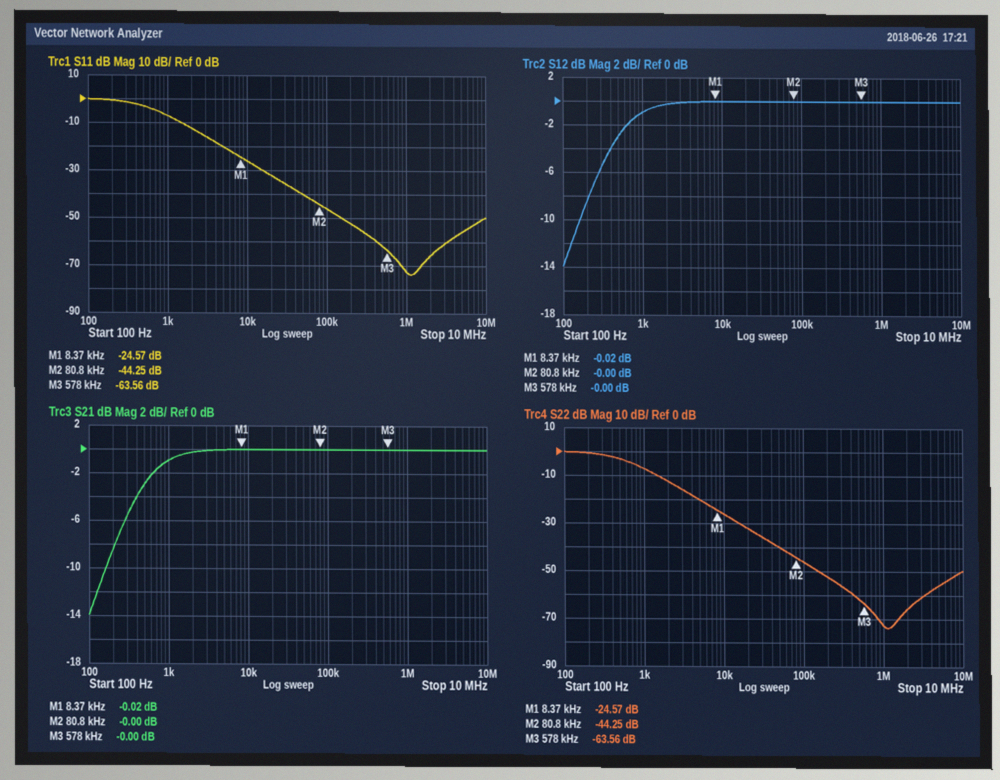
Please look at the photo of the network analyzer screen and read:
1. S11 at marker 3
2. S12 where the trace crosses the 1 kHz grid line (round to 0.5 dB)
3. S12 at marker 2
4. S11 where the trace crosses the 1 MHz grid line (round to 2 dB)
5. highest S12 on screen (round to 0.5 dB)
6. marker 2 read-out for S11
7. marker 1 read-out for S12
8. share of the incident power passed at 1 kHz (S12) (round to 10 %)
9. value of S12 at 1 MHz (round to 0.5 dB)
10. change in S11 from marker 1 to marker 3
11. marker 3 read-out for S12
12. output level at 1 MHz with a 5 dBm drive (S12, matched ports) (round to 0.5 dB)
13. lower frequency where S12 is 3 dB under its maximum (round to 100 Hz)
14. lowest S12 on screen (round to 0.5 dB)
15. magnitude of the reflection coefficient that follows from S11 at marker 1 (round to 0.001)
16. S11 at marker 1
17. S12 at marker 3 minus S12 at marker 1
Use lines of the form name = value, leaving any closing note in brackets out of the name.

S11 at marker 3 = -63.56 dB
S12 where the trace crosses the 1 kHz grid line = -1.0 dB
S12 at marker 2 = -0.00 dB
S11 where the trace crosses the 1 MHz grid line = -72 dB
highest S12 on screen = 0.0 dB
marker 2 read-out for S11 = -44.25 dB
marker 1 read-out for S12 = -0.02 dB
share of the incident power passed at 1 kHz (S12) = 80 %
value of S12 at 1 MHz = 0.0 dB
change in S11 from marker 1 to marker 3 = -38.99 dB
marker 3 read-out for S12 = -0.00 dB
output level at 1 MHz with a 5 dBm drive (S12, matched ports) = 5.0 dBm
lower frequency where S12 is 3 dB under its maximum = 500 Hz
lowest S12 on screen = -14.0 dB
magnitude of the reflection coefficient that follows from S11 at marker 1 = 0.059
S11 at marker 1 = -24.57 dB
S12 at marker 3 minus S12 at marker 1 = 0.02 dB
